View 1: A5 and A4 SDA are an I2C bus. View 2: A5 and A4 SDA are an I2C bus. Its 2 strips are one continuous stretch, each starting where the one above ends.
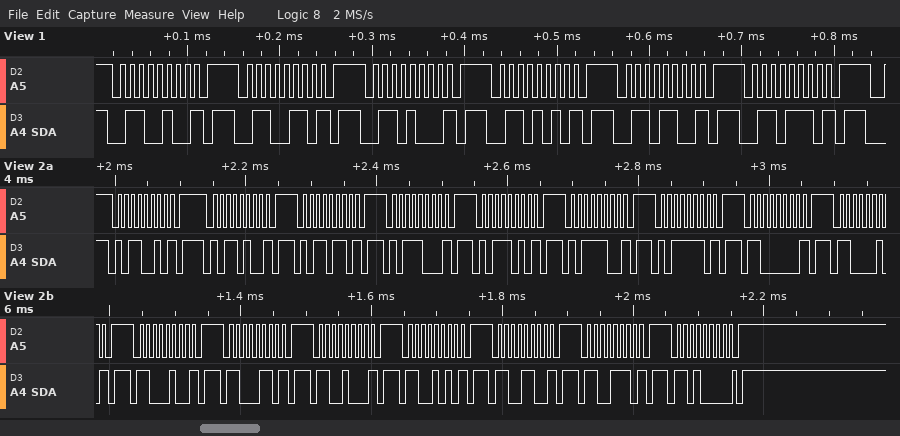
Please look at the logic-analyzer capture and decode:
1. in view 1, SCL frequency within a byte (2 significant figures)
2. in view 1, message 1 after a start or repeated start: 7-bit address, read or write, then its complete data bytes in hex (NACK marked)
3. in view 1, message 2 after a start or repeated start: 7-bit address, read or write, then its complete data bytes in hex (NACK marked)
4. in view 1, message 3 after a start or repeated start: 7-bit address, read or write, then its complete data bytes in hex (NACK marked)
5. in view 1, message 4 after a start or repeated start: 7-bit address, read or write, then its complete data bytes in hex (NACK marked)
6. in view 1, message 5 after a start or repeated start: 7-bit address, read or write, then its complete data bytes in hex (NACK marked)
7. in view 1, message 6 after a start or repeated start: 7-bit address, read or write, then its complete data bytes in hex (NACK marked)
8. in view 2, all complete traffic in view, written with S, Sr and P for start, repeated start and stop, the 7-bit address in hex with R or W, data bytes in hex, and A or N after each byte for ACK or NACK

100 kHz
0x32 write NACK
0x33 write NACK
0x34 write NACK
0x35 write NACK
0x36 write NACK
0x37 write NACK
S 59W N P S 5AW N P S 5BW N P S 5CW N P S 5DW N P S 5EW N P S 5FW N P S 60W N P S 61W N P S 62W N P S 63W N P S 64W N P S 65W N P S 66W N P S 67W N P S 68W A P
